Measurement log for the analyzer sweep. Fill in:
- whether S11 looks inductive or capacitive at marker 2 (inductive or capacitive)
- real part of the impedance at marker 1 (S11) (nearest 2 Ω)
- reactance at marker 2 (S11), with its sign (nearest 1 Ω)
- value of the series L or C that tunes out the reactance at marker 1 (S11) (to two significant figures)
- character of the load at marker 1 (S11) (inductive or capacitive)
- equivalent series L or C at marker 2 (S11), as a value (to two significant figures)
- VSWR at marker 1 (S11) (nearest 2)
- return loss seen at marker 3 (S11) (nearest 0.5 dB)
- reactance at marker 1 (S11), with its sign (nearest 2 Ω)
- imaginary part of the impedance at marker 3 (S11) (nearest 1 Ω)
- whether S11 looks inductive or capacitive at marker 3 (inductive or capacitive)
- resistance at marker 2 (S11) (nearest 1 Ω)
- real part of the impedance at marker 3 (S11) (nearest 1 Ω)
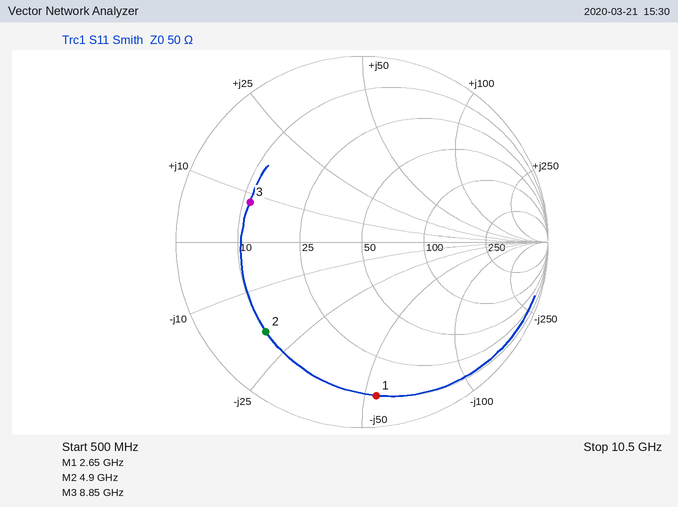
capacitive
10 Ω
-19 Ω
3.2 nH
capacitive
1.7 pF
10
4.0 dB
-54 Ω
+8 Ω
inductive
10 Ω
11 Ω
